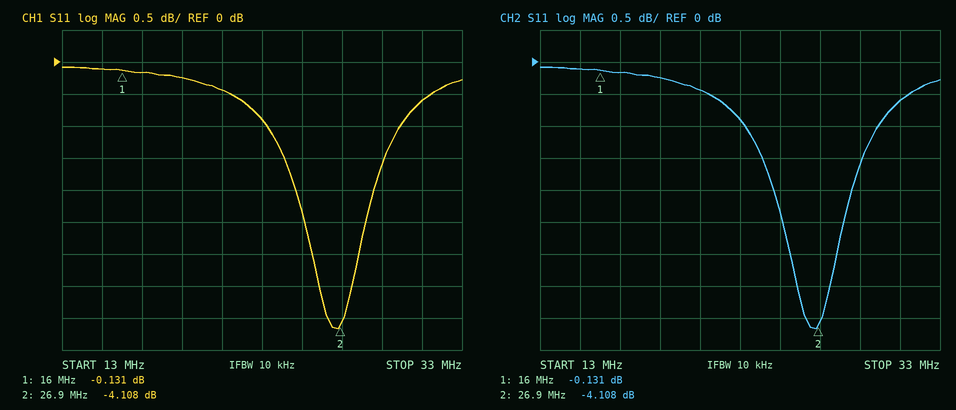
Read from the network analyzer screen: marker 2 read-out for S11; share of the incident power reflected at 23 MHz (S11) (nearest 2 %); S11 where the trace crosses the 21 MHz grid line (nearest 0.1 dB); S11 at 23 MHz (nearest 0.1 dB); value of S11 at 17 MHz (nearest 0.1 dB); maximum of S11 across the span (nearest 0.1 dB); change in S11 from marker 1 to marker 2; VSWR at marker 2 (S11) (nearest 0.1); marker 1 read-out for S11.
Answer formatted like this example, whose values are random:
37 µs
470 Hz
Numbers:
-4.108 dB
82 %
-0.4 dB
-0.9 dB
-0.2 dB
-0.1 dB
-3.977 dB
4.3
-0.131 dB
